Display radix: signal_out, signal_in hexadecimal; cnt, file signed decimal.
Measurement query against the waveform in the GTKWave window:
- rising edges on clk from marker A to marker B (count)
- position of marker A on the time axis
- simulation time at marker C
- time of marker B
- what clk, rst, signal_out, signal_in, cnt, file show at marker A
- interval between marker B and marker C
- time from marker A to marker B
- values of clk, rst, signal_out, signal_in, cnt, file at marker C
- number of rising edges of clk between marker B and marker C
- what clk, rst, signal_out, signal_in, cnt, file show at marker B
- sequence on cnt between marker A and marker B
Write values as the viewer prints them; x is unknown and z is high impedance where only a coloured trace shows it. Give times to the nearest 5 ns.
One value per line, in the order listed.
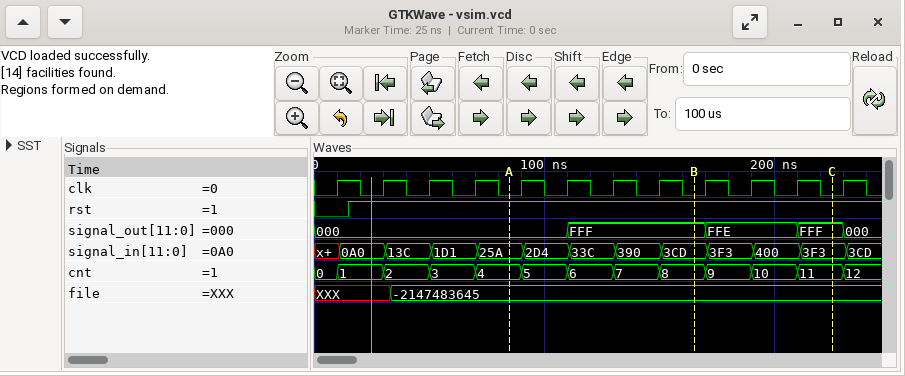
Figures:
4
85 ns
225 ns
165 ns
clk=0, rst=1, signal_out=000, signal_in=25A, cnt=4, file=-2147483645
60 ns
80 ns
clk=0, rst=1, signal_out=FFF, signal_in=3F3, cnt=11, file=-2147483645
3
clk=0, rst=1, signal_out=FFF, signal_in=3CD, cnt=8, file=-2147483645
4, 5, 6, 7, 8
